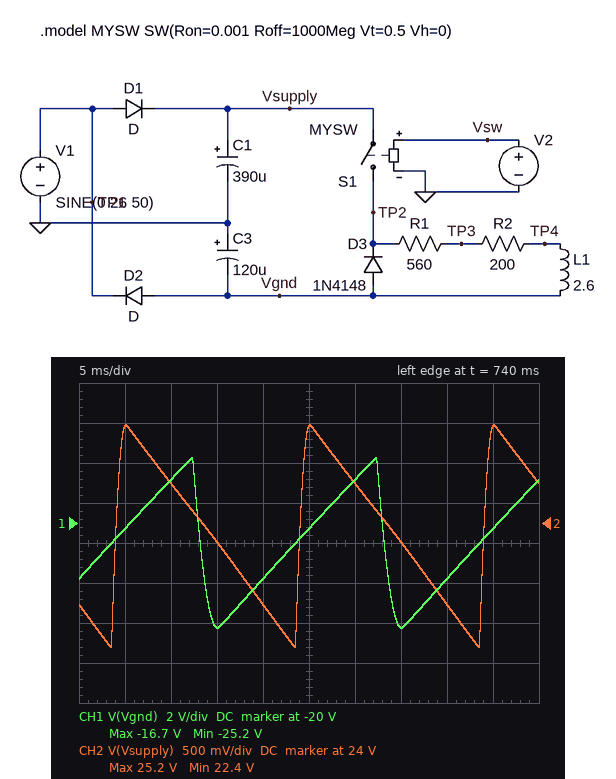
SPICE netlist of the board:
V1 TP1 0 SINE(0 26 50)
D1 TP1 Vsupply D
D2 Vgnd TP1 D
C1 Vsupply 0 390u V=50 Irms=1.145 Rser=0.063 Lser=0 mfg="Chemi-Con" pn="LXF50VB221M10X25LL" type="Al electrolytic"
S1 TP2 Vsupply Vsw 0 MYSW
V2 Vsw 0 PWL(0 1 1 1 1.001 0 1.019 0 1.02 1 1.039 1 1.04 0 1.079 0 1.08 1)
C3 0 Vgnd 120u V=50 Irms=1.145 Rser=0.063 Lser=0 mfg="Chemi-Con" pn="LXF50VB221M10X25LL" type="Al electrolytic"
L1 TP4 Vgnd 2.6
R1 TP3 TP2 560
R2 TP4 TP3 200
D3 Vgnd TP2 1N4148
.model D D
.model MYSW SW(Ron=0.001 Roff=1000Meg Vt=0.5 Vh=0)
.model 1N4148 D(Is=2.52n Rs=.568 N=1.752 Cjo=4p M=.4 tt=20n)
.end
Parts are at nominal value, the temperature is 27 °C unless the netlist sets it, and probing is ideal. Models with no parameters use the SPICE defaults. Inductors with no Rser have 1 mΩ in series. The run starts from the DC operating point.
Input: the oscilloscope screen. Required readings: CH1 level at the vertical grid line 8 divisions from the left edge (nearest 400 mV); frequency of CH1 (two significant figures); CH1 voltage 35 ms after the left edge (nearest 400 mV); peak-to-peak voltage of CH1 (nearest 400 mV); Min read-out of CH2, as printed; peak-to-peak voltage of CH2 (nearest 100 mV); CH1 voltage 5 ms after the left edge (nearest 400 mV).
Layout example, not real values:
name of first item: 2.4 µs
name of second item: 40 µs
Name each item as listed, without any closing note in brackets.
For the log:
CH1 level at the vertical grid line 8 divisions from the left edge: -22.8 V
frequency of CH1: 50 Hz
CH1 voltage 35 ms after the left edge: -25.2 V
peak-to-peak voltage of CH1: 8.4 V
Min read-out of CH2, as printed: 22.4 V
peak-to-peak voltage of CH2: 2.8 V
CH1 voltage 5 ms after the left edge: -20.4 V
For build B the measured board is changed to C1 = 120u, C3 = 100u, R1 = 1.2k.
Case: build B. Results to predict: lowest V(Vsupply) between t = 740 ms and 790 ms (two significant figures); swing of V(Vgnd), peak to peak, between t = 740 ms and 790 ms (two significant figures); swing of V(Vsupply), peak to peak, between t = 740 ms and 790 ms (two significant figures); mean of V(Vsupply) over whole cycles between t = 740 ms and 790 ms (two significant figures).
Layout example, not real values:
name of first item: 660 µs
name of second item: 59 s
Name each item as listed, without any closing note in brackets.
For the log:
lowest V(Vsupply) between t = 740 ms and 790 ms: 20 V
swing of V(Vgnd), peak to peak, between t = 740 ms and 790 ms: 5.7 V
swing of V(Vsupply), peak to peak, between t = 740 ms and 790 ms: 4.8 V
mean of V(Vsupply) over whole cycles between t = 740 ms and 790 ms: 23 V
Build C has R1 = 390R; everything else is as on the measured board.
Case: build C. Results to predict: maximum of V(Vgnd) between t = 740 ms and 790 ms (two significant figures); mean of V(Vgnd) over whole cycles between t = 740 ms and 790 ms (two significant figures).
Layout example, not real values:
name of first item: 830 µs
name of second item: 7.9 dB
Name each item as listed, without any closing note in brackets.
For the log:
maximum of V(Vgnd) between t = 740 ms and 790 ms: -15 V
mean of V(Vgnd) over whole cycles between t = 740 ms and 790 ms: -20 V
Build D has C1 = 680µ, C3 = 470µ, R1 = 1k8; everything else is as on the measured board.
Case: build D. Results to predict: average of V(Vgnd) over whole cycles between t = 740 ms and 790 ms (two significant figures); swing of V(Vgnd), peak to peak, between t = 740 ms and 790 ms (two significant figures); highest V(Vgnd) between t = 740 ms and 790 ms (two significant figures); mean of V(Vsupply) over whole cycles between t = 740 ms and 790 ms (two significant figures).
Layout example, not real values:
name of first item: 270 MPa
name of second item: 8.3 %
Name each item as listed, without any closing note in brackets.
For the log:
average of V(Vgnd) over whole cycles between t = 740 ms and 790 ms: -25 V
swing of V(Vgnd), peak to peak, between t = 740 ms and 790 ms: 1.0 V
highest V(Vgnd) between t = 740 ms and 790 ms: -24 V
mean of V(Vsupply) over whole cycles between t = 740 ms and 790 ms: 25 V
